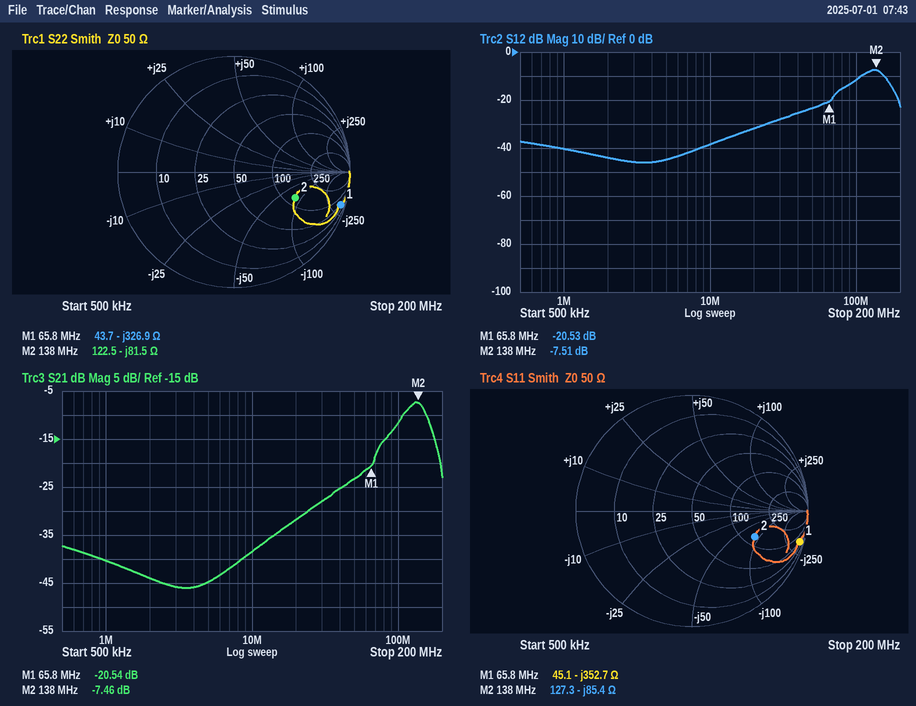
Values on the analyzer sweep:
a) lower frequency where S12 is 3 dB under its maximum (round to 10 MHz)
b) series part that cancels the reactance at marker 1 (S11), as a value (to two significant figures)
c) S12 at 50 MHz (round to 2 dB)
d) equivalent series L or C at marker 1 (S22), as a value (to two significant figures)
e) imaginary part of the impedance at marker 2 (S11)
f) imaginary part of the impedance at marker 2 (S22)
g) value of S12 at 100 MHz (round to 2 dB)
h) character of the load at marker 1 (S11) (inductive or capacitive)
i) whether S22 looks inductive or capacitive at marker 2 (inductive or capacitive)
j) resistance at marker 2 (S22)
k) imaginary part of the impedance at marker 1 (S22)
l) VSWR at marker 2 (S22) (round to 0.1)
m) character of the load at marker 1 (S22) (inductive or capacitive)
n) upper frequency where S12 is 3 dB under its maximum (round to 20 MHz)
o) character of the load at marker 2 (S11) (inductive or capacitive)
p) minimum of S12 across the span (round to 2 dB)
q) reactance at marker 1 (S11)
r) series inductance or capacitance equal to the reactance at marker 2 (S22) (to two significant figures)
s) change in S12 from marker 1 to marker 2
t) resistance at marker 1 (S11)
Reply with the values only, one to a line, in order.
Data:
110 MHz
850 nH
-24 dB
7.4 pF
-85.4 Ω
-81.5 Ω
-12 dB
capacitive
capacitive
122.5 Ω
-326.9 Ω
3.7
capacitive
160 MHz
capacitive
-46 dB
-352.7 Ω
14 pF
13.02 dB
45.1 Ω
